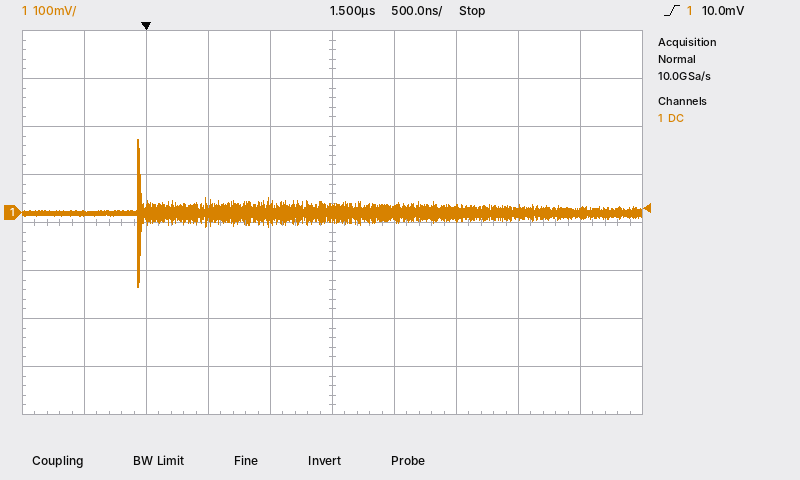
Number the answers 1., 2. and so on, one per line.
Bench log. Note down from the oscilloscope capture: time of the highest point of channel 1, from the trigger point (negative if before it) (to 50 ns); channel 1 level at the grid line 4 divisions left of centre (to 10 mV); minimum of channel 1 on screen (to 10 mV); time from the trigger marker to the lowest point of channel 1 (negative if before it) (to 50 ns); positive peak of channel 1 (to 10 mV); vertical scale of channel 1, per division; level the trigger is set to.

1. -50 ns
2. 0 mV
3. -150 mV
4. -50 ns
5. 150 mV
6. 100 mV
7. 10.0 mV
